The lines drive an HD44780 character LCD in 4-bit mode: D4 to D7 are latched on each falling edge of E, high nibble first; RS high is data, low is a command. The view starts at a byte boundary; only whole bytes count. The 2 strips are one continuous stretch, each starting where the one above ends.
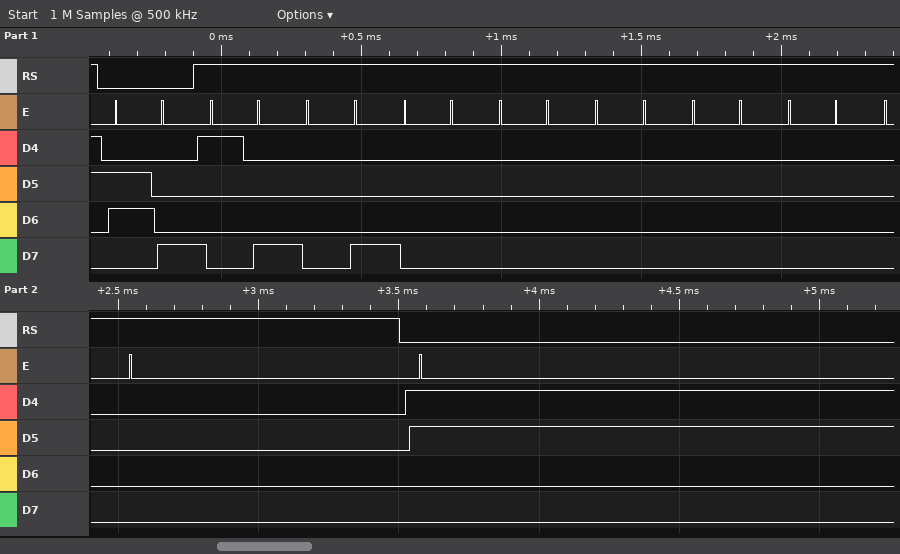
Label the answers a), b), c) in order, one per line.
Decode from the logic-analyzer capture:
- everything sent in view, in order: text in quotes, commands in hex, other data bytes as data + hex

a) 0x68 data 18 08 00 00 00 00 00 00
